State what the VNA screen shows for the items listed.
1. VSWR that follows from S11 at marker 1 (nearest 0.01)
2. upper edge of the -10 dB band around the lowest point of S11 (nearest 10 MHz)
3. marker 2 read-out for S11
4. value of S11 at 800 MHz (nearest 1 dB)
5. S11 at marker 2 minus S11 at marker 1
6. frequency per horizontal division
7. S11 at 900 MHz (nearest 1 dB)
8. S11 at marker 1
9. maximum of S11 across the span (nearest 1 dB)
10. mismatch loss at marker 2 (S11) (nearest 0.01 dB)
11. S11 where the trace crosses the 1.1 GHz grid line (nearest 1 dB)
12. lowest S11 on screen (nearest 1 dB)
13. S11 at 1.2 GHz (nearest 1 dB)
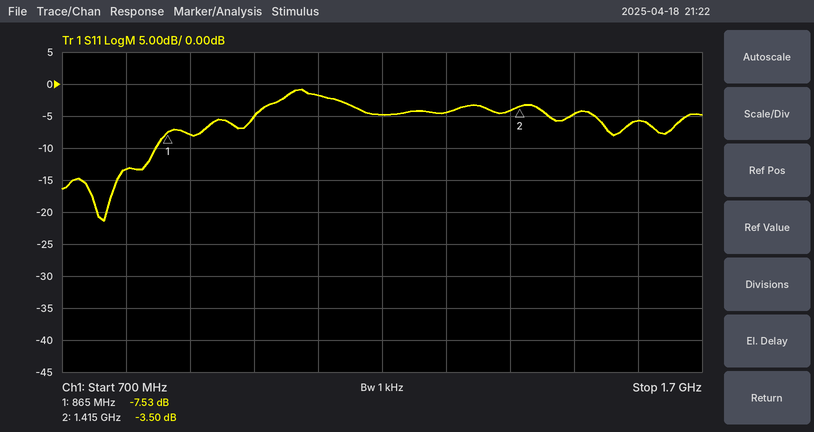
2.45
850 MHz
-3.50 dB
-13 dB
4.03 dB
100 MHz
-8 dB
-7.53 dB
-1 dB
2.57 dB
-2 dB
-21 dB
-5 dB
